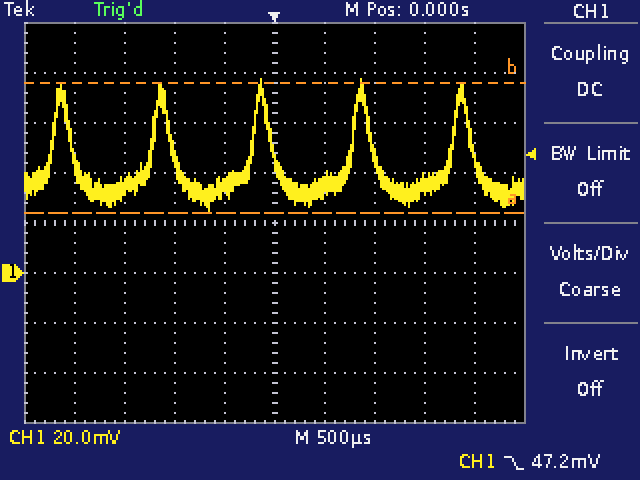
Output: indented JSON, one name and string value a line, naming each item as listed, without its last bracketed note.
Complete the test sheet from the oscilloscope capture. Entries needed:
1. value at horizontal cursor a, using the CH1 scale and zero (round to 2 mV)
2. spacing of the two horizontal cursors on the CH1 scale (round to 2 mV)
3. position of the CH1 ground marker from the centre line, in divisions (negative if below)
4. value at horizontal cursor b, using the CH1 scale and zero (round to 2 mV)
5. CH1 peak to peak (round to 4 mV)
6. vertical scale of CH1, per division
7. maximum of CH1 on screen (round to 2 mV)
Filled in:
{
  "value at horizontal cursor a, using the CH1 scale and zero": "24 mV",
  "spacing of the two horizontal cursors on the CH1 scale": "52 mV",
  "position of the CH1 ground marker from the centre line, in divisions": "-1.0 div",
  "value at horizontal cursor b, using the CH1 scale and zero": "76 mV",
  "CH1 peak to peak": "52 mV",
  "vertical scale of CH1, per division": "20 mV",
  "maximum of CH1 on screen": "78 mV"
}
